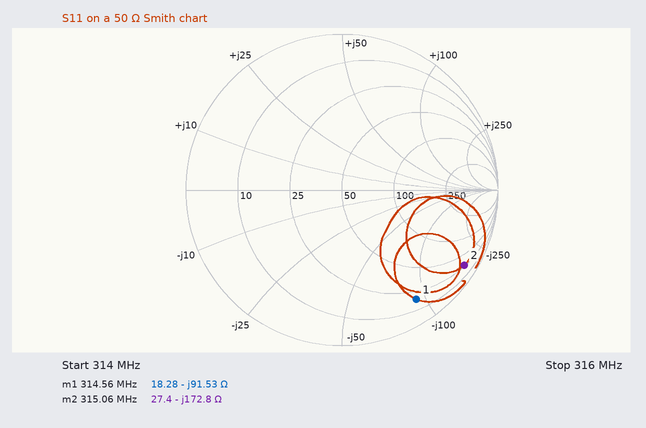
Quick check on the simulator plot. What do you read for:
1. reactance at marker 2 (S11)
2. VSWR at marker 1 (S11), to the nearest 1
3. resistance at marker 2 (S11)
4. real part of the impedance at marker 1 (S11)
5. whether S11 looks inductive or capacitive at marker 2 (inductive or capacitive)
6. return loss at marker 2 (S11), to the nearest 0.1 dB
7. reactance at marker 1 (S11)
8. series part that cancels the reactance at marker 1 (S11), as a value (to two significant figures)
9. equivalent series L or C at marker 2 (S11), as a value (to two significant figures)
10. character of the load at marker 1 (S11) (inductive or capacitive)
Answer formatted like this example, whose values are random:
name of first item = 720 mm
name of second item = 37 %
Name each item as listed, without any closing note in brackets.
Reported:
reactance at marker 2 = -172.8 Ω
VSWR at marker 1 (S11), to the nearest 1 = 12
resistance at marker 2 = 27.4 Ω
real part of the impedance at marker 1 = 18.28 Ω
whether S11 looks inductive or capacitive at marker 2 = capacitive
return loss at marker 2 (S11), to the nearest 0.1 dB = 0.7 dB
reactance at marker 1 = -91.53 Ω
series part that cancels the reactance at marker 1 (S11), as a value = 46 nH
equivalent series L or C at marker 2 (S11), as a value = 2.9 pF
character of the load at marker 1 (S11) = capacitive
